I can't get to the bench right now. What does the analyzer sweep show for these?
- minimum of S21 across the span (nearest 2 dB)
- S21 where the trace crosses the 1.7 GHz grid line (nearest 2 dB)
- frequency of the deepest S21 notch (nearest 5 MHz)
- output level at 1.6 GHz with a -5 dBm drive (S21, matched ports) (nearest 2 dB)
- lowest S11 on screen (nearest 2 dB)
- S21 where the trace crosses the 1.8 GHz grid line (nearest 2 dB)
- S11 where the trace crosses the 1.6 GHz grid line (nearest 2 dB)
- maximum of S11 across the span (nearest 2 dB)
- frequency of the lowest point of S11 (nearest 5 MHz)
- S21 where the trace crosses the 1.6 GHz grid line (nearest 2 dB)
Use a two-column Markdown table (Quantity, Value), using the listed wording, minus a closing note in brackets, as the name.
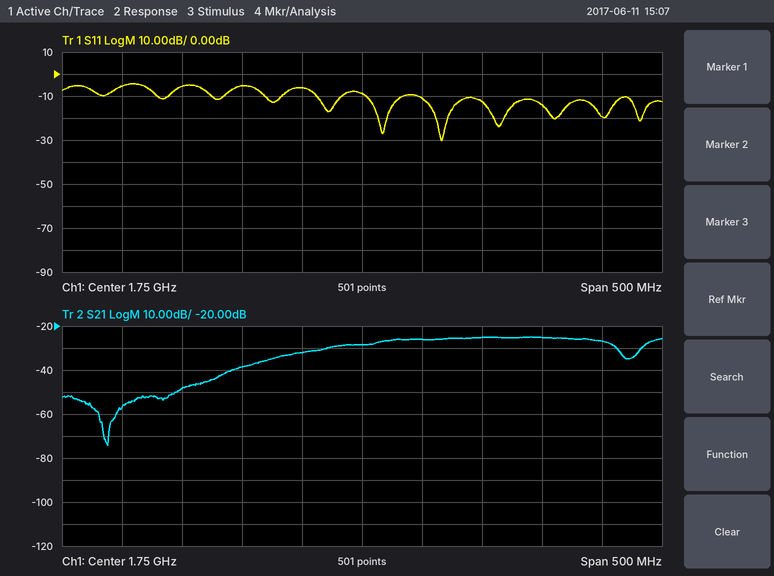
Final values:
| Quantity | Value |
|---|---|
| minimum of S21 across the span | -74 dB |
| S21 where the trace crosses the 1.7 GHz grid line | -32 dB |
| frequency of the deepest S21 notch | 1.540 GHz |
| output level at 1.6 GHz with a -5 dBm drive (S21, matched ports) | -54 dBm |
| lowest S11 on screen | -30 dB |
| S21 where the trace crosses the 1.8 GHz grid line | -26 dB |
| S11 where the trace crosses the 1.6 GHz grid line | -6 dB |
| maximum of S11 across the span | -4 dB |
| frequency of the lowest point of S11 | 1.815 GHz |
| S21 where the trace crosses the 1.6 GHz grid line | -48 dB |
